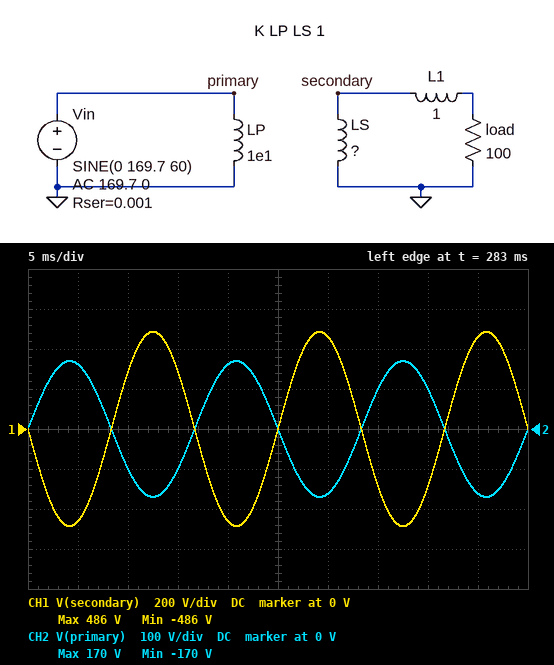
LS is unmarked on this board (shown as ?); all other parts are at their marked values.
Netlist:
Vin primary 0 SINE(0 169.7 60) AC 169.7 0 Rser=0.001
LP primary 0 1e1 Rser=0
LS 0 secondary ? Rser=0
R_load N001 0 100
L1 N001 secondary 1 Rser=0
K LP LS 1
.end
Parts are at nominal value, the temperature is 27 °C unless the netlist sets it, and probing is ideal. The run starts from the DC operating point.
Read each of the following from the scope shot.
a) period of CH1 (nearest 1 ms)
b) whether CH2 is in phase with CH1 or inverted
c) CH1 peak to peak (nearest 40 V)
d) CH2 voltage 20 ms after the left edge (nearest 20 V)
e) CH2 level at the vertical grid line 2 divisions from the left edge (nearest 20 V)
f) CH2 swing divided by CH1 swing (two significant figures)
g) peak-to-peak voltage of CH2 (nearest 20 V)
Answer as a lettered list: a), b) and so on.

a) 17 ms
b) inverted
c) 960 V
d) 160 V
e) -100 V
f) 0.35
g) 340 V
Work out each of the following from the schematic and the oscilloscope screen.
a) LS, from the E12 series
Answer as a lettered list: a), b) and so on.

a) 82 H
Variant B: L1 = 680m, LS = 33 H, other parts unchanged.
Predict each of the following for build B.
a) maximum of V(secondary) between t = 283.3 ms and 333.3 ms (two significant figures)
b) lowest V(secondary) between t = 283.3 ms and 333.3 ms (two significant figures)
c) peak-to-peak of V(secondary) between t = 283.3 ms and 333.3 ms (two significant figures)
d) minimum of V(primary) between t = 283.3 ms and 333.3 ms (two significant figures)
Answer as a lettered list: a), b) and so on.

a) 310 V
b) -310 V
c) 620 V
d) -170 V
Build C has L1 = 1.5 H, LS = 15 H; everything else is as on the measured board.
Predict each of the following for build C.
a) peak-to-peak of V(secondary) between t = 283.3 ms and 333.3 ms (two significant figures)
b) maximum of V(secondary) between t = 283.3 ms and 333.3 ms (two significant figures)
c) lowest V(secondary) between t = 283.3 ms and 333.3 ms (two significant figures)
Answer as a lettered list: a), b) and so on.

a) 420 V
b) 210 V
c) -210 V
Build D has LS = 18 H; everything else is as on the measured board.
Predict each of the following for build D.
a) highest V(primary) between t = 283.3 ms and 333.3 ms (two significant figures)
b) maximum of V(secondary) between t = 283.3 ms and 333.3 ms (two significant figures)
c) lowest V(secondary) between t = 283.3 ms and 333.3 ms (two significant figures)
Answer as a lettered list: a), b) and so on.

a) 170 V
b) 230 V
c) -230 V
